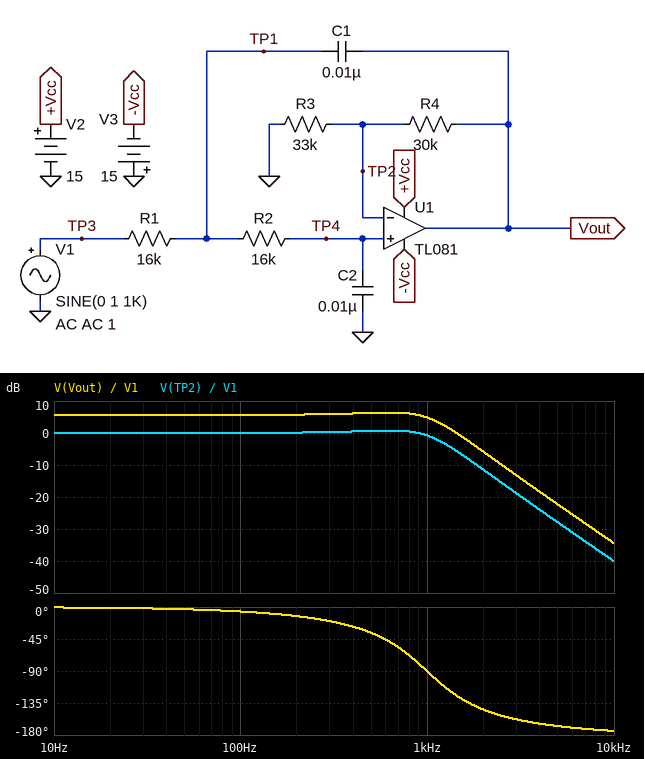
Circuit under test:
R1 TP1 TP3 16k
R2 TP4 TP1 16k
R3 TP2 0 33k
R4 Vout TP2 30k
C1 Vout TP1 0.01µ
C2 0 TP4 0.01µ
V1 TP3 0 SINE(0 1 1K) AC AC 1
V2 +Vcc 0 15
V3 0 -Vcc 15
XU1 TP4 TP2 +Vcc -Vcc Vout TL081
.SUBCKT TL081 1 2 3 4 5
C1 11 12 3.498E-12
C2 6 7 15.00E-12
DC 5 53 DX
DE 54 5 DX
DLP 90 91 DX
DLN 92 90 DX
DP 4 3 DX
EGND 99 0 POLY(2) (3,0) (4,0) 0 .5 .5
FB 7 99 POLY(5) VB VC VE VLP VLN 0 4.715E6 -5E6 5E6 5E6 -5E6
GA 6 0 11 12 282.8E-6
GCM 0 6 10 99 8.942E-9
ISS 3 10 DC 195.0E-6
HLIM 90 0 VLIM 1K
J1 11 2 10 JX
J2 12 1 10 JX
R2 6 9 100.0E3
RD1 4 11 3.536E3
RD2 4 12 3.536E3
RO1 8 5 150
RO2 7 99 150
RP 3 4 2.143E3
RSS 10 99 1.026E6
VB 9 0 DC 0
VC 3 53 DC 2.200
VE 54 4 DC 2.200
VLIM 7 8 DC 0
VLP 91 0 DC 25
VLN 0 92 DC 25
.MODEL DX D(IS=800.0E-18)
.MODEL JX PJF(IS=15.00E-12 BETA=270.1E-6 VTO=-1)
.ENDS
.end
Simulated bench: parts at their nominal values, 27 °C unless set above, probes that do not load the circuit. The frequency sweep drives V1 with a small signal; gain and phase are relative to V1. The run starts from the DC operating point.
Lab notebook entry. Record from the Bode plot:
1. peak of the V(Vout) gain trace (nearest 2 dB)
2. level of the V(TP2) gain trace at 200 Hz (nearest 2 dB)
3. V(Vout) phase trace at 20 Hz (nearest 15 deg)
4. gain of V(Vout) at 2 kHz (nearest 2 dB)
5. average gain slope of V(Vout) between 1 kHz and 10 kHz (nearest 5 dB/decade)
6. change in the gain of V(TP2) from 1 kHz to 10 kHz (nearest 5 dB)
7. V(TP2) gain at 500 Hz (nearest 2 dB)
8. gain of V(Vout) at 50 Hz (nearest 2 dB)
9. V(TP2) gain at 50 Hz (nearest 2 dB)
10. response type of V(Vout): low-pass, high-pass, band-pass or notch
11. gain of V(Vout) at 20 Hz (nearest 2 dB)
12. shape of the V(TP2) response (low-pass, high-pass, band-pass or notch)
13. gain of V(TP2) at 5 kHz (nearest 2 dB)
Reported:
6 dB
0 dB
0 deg
-6 dB
-40 dB/decade
-40 dB
0 dB
6 dB
0 dB
low-pass
6 dB
low-pass
-28 dB
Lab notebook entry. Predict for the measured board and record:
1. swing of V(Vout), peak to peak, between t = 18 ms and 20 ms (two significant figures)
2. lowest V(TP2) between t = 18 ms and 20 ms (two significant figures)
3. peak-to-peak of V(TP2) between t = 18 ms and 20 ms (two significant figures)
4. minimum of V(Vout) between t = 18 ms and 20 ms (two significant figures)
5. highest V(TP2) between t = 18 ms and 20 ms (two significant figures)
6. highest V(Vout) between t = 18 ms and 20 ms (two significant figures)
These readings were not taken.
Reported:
3.5 V
-910 mV
1.8 V
-1.7 V
910 mV
1.7 V
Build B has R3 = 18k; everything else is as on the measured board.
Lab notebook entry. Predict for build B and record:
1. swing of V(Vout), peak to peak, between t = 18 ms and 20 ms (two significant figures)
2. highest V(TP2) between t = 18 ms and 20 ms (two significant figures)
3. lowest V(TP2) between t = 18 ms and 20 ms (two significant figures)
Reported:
16 V
3.0 V
-3.0 V
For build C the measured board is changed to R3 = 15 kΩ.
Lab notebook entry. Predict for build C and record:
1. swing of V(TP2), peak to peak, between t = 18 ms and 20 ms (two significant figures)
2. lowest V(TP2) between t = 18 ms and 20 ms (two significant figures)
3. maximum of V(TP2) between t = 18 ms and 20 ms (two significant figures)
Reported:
9.0 V
-4.5 V
4.5 V
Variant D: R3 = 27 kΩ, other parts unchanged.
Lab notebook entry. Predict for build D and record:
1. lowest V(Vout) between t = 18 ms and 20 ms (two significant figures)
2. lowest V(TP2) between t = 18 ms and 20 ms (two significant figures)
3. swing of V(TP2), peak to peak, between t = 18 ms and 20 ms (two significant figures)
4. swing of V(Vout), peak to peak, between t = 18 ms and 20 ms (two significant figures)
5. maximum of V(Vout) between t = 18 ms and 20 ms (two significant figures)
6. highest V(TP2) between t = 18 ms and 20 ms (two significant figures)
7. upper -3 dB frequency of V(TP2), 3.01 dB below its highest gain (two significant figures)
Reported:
-2.4 V
-1.1 V
2.2 V
4.7 V
2.4 V
1.1 V
1.2 kHz
